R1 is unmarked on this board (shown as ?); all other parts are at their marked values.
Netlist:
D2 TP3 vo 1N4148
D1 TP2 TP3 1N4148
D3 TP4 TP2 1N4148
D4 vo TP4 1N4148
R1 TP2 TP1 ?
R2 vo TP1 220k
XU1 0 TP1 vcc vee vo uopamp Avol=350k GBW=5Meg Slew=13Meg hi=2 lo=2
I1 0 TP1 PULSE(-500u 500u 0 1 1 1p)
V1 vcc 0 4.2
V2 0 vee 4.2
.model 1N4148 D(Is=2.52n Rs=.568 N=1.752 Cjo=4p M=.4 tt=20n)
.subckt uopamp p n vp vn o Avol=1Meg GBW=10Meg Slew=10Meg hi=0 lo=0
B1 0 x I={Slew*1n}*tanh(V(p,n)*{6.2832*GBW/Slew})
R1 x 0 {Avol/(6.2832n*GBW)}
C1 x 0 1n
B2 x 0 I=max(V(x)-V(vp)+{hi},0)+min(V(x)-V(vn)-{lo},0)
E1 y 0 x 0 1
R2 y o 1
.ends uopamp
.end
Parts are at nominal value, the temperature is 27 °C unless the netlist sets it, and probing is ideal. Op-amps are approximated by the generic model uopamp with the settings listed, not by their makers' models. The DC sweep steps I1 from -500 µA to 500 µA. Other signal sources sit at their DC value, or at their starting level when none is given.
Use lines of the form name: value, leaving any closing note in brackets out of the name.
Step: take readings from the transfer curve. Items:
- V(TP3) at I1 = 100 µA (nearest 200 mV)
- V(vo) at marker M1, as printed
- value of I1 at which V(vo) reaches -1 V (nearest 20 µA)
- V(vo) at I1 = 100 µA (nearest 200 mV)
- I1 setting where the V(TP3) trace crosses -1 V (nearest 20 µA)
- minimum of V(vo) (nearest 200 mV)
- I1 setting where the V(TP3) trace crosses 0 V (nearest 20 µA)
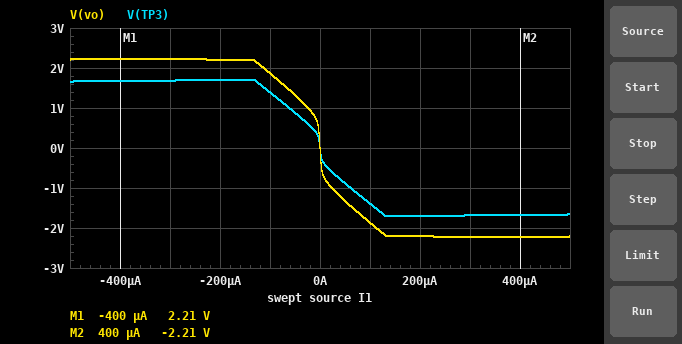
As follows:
V(TP3) at I1 = 100 µA: -1.4 V
V(vo) at marker M1, as printed: 2.21 V
value of I1 at which V(vo) reaches -1 V: 20 µA
V(vo) at I1 = 100 µA: -1.8 V
I1 setting where the V(TP3) trace crosses -1 V: 60 µA
minimum of V(vo): -2.2 V
I1 setting where the V(TP3) trace crosses 0 V: 0 A
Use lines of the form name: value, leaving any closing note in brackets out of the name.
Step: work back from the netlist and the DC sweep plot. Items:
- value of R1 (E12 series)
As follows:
value of R1: 10 kΩ
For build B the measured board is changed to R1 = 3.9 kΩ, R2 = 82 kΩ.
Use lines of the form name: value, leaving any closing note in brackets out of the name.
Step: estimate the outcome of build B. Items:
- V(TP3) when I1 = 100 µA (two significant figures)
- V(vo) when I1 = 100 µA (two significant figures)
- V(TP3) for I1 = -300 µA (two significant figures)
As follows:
V(TP3) when I1 = 100 µA: -800 mV
V(vo) when I1 = 100 µA: -1.3 V
V(TP3) for I1 = -300 µA: 1.6 V
